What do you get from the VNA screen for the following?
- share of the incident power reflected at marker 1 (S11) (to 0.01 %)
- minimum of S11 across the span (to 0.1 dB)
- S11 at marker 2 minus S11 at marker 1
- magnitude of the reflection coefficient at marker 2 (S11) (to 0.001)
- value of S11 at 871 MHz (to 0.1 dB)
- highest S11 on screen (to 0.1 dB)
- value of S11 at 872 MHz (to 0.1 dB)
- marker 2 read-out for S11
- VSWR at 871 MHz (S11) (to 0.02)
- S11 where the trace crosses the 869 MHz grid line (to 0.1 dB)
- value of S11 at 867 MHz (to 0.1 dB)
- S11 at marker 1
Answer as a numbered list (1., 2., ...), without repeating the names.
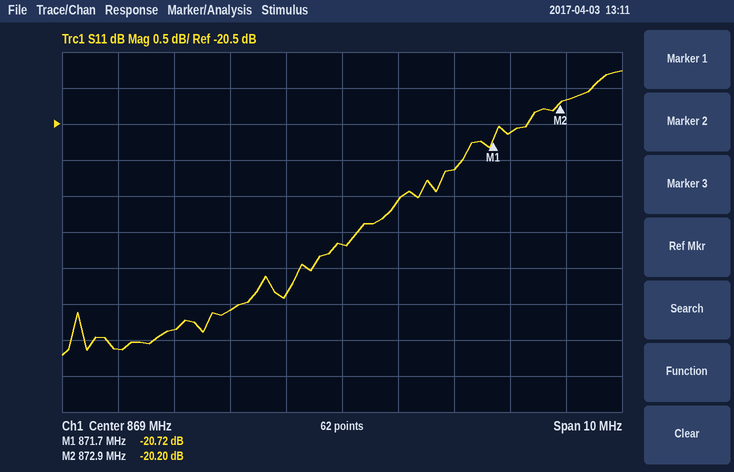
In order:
1. 0.85 %
2. -23.7 dB
3. 0.52 dB
4. 0.098
5. -21.1 dB
6. -19.8 dB
7. -20.6 dB
8. -20.20 dB
9. 1.20
10. -22.2 dB
11. -23.1 dB
12. -20.72 dB
